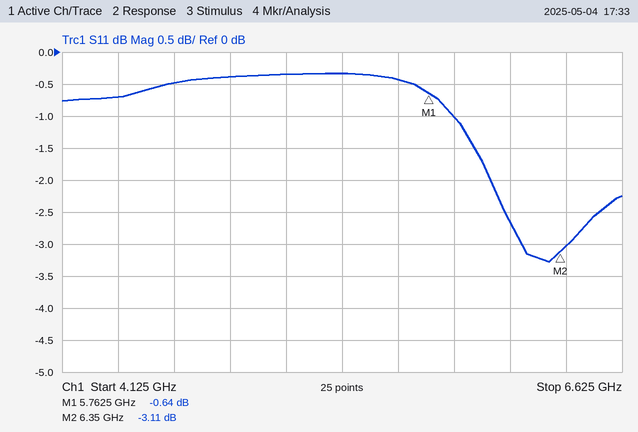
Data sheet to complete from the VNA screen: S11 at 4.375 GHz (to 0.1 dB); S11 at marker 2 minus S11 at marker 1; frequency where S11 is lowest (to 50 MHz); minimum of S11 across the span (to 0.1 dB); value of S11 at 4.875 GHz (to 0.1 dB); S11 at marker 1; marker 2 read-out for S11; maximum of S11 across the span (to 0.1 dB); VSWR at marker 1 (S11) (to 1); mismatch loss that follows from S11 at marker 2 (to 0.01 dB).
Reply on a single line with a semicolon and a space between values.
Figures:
-0.7 dB; -2.47 dB; 6.30 GHz; -3.3 dB; -0.4 dB; -0.64 dB; -3.11 dB; -0.3 dB; 27; 2.91 dB
